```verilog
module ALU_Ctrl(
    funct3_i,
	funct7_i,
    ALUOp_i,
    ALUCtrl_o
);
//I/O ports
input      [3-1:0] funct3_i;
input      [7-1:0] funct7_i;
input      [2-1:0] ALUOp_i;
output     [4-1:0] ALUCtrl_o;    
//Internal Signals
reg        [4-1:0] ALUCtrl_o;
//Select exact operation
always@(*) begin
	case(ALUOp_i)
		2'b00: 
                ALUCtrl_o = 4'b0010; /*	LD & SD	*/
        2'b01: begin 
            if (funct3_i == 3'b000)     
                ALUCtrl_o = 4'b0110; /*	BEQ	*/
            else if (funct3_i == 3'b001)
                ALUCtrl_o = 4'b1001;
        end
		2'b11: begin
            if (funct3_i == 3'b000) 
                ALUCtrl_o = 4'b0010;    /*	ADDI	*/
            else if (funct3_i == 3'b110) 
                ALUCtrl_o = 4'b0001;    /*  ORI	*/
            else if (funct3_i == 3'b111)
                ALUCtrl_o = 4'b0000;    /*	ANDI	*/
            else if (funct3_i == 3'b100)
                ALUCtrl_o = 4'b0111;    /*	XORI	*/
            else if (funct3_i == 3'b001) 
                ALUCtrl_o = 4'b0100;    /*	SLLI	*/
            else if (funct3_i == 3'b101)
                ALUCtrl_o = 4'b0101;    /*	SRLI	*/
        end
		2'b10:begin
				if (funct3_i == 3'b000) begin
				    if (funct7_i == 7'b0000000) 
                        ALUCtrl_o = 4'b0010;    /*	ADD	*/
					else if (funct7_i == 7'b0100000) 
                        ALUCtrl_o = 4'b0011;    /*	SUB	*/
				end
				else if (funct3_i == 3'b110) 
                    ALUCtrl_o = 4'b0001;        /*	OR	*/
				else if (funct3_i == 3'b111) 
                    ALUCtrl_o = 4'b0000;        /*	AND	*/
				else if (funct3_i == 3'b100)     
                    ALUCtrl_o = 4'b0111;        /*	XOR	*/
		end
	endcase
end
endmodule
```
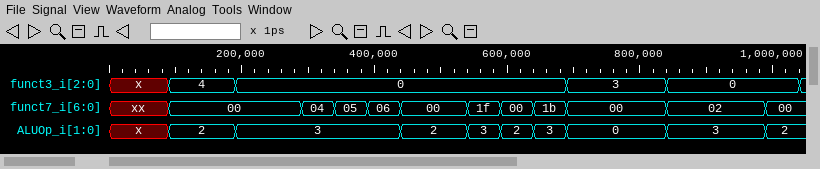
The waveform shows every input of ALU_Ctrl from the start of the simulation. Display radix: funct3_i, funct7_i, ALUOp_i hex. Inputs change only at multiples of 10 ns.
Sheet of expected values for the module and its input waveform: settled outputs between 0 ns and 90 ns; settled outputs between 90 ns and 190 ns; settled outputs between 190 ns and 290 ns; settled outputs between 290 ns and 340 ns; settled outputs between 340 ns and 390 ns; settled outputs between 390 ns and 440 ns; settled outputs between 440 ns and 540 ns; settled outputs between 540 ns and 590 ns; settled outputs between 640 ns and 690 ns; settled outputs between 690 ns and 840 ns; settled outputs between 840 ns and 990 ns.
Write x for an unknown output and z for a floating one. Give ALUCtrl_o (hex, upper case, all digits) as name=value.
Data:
ALUCtrl_o=x
ALUCtrl_o=7
ALUCtrl_o=2
ALUCtrl_o=2
ALUCtrl_o=2
ALUCtrl_o=2
ALUCtrl_o=2
ALUCtrl_o=2
ALUCtrl_o=2
ALUCtrl_o=2
ALUCtrl_o=2
